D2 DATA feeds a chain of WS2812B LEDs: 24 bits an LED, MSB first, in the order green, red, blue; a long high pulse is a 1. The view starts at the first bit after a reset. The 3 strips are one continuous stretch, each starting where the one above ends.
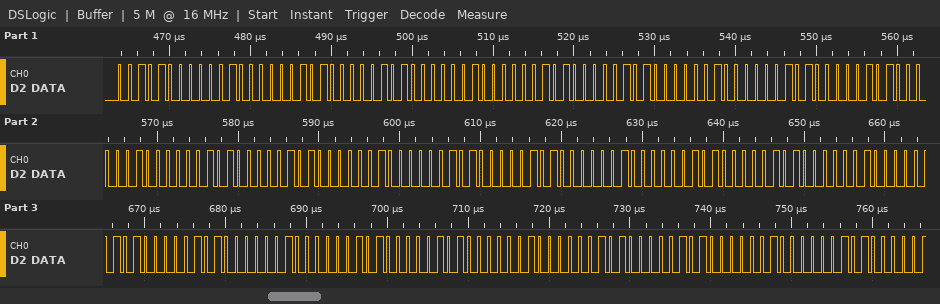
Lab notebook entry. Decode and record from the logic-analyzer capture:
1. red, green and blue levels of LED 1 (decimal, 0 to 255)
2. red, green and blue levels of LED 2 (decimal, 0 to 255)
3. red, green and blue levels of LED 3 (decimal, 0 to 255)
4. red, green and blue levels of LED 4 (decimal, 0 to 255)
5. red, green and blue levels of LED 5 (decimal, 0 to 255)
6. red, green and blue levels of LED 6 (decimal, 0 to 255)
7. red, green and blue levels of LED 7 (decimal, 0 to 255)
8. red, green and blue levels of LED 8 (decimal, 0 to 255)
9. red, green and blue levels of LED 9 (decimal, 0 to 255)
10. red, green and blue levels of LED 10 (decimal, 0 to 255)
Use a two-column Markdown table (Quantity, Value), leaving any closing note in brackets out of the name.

| Quantity | Value |
|---|---|
| red, green and blue levels of LED 1 | 16, 40, 40 |
| red, green and blue levels of LED 2 | 16, 40, 40 |
| red, green and blue levels of LED 3 | 16, 40, 40 |
| red, green and blue levels of LED 4 | 16, 40, 40 |
| red, green and blue levels of LED 5 | 16, 40, 40 |
| red, green and blue levels of LED 6 | 16, 40, 40 |
| red, green and blue levels of LED 7 | 16, 40, 40 |
| red, green and blue levels of LED 8 | 16, 40, 40 |
| red, green and blue levels of LED 9 | 16, 40, 40 |
| red, green and blue levels of LED 10 | 16, 40, 40 |
